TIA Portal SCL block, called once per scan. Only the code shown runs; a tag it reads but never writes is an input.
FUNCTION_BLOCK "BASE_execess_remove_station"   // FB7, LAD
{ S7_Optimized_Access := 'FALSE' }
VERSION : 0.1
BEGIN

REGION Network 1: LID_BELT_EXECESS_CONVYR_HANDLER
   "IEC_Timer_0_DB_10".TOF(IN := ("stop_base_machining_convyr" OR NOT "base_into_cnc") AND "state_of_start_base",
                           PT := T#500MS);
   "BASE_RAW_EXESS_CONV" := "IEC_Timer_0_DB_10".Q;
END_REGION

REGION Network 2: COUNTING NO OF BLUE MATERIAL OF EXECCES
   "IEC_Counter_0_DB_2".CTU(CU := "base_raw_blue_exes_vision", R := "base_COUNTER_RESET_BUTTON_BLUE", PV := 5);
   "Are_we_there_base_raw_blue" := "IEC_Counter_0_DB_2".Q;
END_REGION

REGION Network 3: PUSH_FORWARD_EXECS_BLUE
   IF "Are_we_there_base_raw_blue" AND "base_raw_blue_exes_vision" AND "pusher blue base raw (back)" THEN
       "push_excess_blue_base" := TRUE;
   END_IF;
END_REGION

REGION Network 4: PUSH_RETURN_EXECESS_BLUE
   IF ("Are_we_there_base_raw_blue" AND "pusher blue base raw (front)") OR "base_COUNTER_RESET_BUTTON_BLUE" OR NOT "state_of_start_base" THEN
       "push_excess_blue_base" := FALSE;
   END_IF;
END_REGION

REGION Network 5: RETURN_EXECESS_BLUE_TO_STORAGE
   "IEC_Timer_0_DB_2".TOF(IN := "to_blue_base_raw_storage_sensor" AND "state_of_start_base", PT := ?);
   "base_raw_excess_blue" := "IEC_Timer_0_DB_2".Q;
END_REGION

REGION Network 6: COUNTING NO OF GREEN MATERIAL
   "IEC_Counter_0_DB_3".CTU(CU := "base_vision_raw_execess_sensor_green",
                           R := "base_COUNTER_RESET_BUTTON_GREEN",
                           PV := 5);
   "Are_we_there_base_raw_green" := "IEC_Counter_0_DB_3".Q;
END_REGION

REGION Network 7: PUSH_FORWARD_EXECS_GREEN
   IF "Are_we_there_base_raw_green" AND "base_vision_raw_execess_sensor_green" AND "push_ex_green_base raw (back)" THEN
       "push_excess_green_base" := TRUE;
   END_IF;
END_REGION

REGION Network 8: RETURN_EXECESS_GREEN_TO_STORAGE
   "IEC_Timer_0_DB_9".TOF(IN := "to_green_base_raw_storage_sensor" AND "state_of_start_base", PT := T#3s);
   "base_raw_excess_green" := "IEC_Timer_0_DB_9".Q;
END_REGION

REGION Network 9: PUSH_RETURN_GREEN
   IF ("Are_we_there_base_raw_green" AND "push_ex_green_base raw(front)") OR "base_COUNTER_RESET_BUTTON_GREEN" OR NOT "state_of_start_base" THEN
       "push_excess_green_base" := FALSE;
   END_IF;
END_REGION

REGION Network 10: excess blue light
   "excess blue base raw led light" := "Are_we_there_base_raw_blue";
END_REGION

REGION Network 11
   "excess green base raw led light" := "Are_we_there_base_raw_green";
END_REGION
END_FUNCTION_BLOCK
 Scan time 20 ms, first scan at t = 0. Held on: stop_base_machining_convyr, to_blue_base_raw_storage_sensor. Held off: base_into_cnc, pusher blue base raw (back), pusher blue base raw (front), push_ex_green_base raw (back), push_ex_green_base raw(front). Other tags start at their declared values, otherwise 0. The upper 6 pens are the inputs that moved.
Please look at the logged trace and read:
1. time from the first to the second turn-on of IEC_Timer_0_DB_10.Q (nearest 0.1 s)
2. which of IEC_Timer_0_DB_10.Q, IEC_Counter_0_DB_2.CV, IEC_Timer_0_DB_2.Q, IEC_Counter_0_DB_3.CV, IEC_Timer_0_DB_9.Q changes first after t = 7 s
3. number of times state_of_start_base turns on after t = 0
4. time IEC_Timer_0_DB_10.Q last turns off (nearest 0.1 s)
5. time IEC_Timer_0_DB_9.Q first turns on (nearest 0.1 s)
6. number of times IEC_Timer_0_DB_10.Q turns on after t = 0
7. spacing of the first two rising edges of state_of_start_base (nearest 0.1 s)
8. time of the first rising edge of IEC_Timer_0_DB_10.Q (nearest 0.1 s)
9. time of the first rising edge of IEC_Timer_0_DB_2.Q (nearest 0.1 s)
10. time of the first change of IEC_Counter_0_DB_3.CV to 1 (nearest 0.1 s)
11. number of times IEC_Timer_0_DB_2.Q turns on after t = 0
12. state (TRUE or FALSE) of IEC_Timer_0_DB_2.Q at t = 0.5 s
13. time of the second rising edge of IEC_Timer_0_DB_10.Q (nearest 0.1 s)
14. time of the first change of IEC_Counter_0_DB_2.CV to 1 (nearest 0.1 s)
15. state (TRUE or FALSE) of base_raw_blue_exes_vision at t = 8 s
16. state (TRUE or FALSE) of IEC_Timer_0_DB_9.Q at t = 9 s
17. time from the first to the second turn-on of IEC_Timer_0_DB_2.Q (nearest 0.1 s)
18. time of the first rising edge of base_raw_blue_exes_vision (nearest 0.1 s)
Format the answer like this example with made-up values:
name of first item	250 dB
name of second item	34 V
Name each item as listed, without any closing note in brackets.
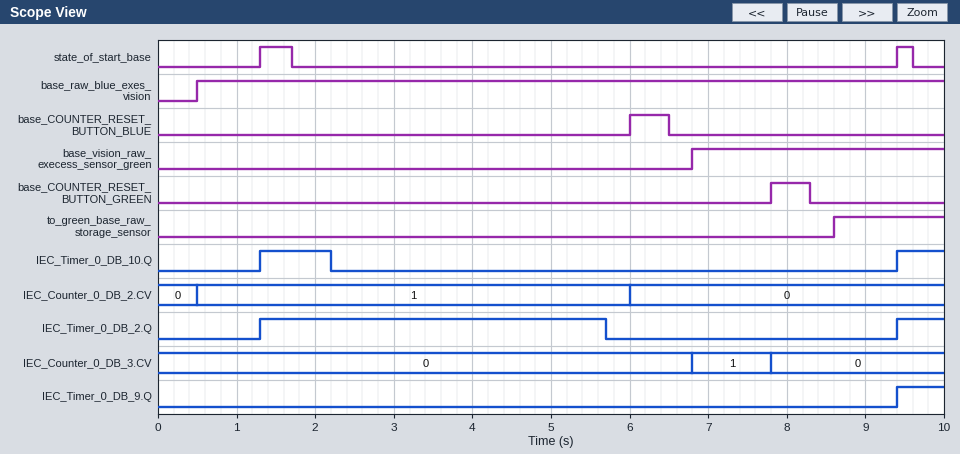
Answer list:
time from the first to the second turn-on of IEC_Timer_0_DB_10.Q	8.1 s
which of IEC_Timer_0_DB_10.Q, IEC_Counter_0_DB_2.CV, IEC_Timer_0_DB_2.Q, IEC_Counter_0_DB_3.CV, IEC_Timer_0_DB_9.Q changes first after t = 7 s	IEC_Counter_0_DB_3.CV
number of times state_of_start_base turns on after t = 0	2
time IEC_Timer_0_DB_10.Q last turns off	2.2 s
time IEC_Timer_0_DB_9.Q first turns on	9.4 s
number of times IEC_Timer_0_DB_10.Q turns on after t = 0	2
spacing of the first two rising edges of state_of_start_base	8.1 s
time of the first rising edge of IEC_Timer_0_DB_10.Q	1.3 s
time of the first rising edge of IEC_Timer_0_DB_2.Q	1.3 s
time of the first change of IEC_Counter_0_DB_3.CV to 1	6.8 s
number of times IEC_Timer_0_DB_2.Q turns on after t = 0	2
state (TRUE or FALSE) of IEC_Timer_0_DB_2.Q at t = 0.5 s	FALSE
time of the second rising edge of IEC_Timer_0_DB_10.Q	9.4 s
time of the first change of IEC_Counter_0_DB_2.CV to 1	0.5 s
state (TRUE or FALSE) of base_raw_blue_exes_vision at t = 8 s	TRUE
state (TRUE or FALSE) of IEC_Timer_0_DB_9.Q at t = 9 s	FALSE
time from the first to the second turn-on of IEC_Timer_0_DB_2.Q	8.1 s
time of the first rising edge of base_raw_blue_exes_vision	0.5 s
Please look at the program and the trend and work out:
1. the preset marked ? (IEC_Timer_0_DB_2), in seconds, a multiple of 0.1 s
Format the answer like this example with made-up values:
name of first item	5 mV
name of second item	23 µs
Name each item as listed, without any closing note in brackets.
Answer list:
the preset marked ? (IEC_Timer_0_DB_2), in seconds, a multiple of 0.1 s	4.0 s
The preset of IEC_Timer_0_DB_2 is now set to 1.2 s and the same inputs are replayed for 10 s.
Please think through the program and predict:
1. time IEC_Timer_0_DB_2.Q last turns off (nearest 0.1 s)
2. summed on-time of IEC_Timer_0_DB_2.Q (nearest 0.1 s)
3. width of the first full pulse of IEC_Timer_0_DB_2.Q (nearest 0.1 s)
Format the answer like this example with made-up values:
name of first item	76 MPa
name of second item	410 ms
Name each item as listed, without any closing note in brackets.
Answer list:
time IEC_Timer_0_DB_2.Q last turns off	2.9 s
summed on-time of IEC_Timer_0_DB_2.Q	2.2 s
width of the first full pulse of IEC_Timer_0_DB_2.Q	1.6 s
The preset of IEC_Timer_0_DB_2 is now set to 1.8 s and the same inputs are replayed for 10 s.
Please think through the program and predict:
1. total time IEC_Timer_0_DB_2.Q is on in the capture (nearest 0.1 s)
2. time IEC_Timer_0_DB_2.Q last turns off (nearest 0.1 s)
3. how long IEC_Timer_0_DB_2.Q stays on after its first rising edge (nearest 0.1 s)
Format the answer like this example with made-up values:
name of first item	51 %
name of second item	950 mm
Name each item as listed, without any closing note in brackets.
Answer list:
total time IEC_Timer_0_DB_2.Q is on in the capture	2.8 s
time IEC_Timer_0_DB_2.Q last turns off	3.5 s
how long IEC_Timer_0_DB_2.Q stays on after its first rising edge	2.2 s
